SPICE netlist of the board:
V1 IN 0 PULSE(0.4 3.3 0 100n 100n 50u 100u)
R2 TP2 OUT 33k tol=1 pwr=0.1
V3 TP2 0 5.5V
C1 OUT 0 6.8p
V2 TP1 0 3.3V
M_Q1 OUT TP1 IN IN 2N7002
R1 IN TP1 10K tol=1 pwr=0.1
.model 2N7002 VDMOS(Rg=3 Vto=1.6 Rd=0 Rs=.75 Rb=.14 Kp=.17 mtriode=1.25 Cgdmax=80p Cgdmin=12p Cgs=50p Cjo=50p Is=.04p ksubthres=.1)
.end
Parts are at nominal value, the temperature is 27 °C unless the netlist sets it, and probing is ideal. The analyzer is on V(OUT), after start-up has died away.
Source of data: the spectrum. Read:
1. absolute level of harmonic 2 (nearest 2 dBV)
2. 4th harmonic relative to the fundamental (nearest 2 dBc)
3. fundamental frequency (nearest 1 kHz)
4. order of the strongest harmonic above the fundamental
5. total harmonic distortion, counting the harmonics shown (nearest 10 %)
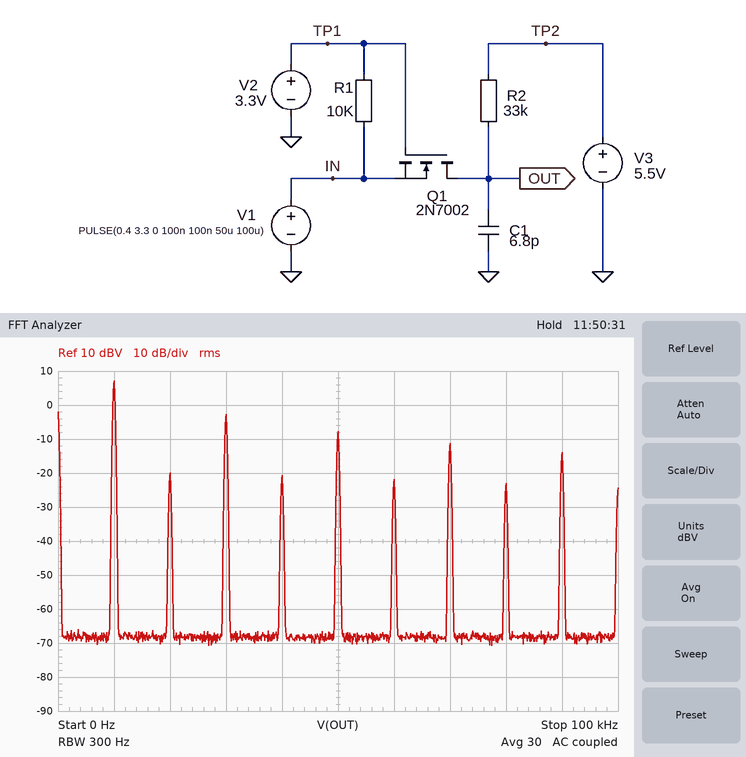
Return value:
-20 dBV
-28 dBc
10 kHz
3
40 %
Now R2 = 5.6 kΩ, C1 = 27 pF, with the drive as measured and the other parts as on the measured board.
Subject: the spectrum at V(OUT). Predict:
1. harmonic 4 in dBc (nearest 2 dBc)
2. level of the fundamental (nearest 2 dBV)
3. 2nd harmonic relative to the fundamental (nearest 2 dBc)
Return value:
-42 dBc
8 dBV
-42 dBc
